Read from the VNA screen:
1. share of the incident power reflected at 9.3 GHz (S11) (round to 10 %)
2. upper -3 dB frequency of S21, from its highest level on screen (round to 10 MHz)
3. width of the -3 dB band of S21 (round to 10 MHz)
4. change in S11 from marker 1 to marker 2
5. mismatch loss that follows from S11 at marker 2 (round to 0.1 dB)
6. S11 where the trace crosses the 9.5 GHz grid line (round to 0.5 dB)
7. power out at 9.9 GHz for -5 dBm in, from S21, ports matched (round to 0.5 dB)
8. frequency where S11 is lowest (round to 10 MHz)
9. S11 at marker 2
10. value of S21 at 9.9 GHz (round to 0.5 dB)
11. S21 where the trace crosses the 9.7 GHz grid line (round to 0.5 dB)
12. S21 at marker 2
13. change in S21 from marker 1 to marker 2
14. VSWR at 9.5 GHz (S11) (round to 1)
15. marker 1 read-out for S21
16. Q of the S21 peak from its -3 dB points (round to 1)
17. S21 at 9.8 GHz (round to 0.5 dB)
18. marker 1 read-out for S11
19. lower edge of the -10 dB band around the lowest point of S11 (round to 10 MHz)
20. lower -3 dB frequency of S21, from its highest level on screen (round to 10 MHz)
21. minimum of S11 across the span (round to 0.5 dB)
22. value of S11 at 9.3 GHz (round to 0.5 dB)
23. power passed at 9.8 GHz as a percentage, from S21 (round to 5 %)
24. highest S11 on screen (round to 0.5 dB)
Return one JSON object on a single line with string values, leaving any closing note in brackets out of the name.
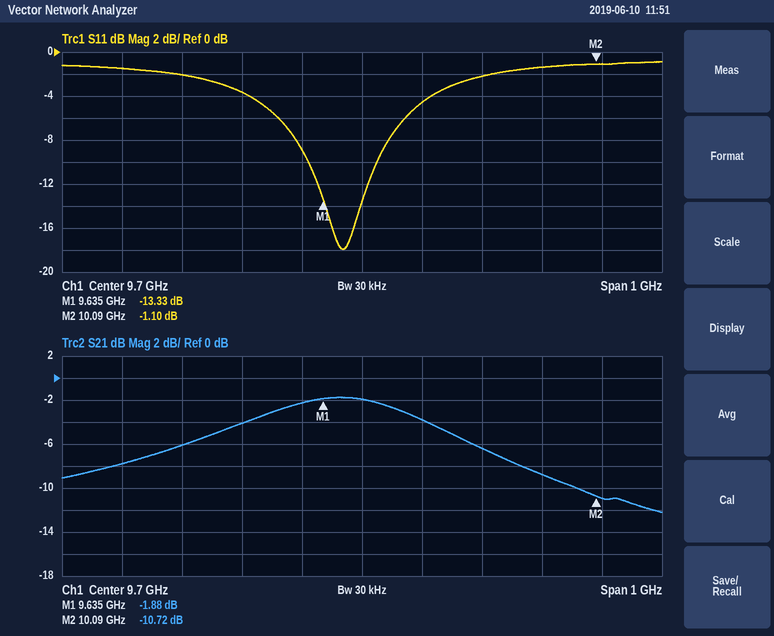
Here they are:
{"share of the incident power reflected at 9.3 GHz (S11)": "70 %", "upper -3 dB frequency of S21, from its highest level on screen": "9.84 GHz", "width of the -3 dB band of S21": "370 MHz", "change in S11 from marker 1 to marker 2": "12.23 dB", "mismatch loss that follows from S11 at marker 2": "6.5 dB", "S11 where the trace crosses the 9.5 GHz grid line": "-3.5 dB", "power out at 9.9 GHz for -5 dBm in, from S21, ports matched": "-11.5 dBm", "frequency where S11 is lowest": "9.67 GHz", "S11 at marker 2": "-1.10 dB", "value of S21 at 9.9 GHz": "-6.5 dB", "S21 where the trace crosses the 9.7 GHz grid line": "-2.0 dB", "S21 at marker 2": "-10.72 dB", "change in S21 from marker 1 to marker 2": "-8.84 dB", "VSWR at 9.5 GHz (S11)": "5", "marker 1 read-out for S21": "-1.88 dB", "Q of the S21 peak from its -3 dB points": "26", "S21 at 9.8 GHz": "-4.0 dB", "marker 1 read-out for S11": "-13.33 dB", "lower edge of the -10 dB band around the lowest point of S11": "9.61 GHz", "lower -3 dB frequency of S21, from its highest level on screen": "9.47 GHz", "minimum of S11 across the span": "-18.0 dB", "value of S11 at 9.3 GHz": "-1.5 dB", "power passed at 9.8 GHz as a percentage, from S21": "40 %", "highest S11 on screen": "-1.0 dB"}
